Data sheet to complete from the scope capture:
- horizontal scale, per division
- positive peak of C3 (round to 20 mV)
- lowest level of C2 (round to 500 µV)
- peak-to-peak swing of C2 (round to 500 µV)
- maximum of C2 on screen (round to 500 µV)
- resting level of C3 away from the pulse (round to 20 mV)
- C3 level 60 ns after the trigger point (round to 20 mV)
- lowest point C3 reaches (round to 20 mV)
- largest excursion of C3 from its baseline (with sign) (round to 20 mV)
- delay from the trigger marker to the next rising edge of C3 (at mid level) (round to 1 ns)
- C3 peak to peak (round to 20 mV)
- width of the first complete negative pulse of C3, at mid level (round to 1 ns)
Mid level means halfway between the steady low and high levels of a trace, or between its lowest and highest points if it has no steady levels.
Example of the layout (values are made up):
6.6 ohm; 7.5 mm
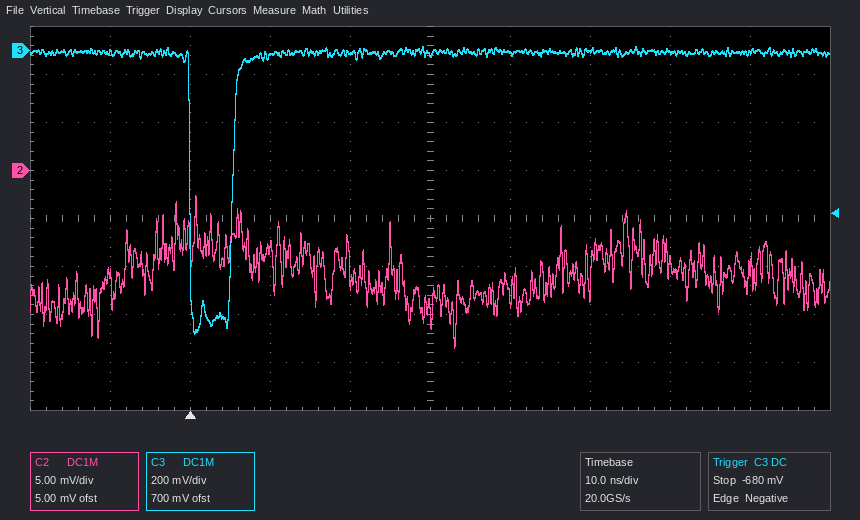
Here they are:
10 ns; 20 mV; -18.5 mV; 16.0 mV; -2.5 mV; 0 mV; 0 mV; -1.18 V; -1.18 V; 5 ns; 1.20 V; 5 ns
